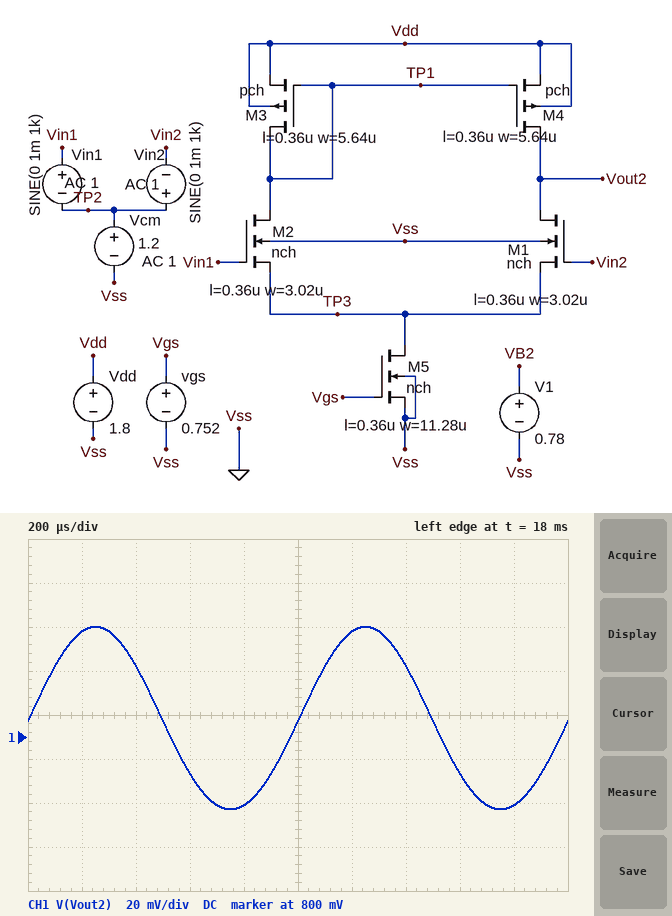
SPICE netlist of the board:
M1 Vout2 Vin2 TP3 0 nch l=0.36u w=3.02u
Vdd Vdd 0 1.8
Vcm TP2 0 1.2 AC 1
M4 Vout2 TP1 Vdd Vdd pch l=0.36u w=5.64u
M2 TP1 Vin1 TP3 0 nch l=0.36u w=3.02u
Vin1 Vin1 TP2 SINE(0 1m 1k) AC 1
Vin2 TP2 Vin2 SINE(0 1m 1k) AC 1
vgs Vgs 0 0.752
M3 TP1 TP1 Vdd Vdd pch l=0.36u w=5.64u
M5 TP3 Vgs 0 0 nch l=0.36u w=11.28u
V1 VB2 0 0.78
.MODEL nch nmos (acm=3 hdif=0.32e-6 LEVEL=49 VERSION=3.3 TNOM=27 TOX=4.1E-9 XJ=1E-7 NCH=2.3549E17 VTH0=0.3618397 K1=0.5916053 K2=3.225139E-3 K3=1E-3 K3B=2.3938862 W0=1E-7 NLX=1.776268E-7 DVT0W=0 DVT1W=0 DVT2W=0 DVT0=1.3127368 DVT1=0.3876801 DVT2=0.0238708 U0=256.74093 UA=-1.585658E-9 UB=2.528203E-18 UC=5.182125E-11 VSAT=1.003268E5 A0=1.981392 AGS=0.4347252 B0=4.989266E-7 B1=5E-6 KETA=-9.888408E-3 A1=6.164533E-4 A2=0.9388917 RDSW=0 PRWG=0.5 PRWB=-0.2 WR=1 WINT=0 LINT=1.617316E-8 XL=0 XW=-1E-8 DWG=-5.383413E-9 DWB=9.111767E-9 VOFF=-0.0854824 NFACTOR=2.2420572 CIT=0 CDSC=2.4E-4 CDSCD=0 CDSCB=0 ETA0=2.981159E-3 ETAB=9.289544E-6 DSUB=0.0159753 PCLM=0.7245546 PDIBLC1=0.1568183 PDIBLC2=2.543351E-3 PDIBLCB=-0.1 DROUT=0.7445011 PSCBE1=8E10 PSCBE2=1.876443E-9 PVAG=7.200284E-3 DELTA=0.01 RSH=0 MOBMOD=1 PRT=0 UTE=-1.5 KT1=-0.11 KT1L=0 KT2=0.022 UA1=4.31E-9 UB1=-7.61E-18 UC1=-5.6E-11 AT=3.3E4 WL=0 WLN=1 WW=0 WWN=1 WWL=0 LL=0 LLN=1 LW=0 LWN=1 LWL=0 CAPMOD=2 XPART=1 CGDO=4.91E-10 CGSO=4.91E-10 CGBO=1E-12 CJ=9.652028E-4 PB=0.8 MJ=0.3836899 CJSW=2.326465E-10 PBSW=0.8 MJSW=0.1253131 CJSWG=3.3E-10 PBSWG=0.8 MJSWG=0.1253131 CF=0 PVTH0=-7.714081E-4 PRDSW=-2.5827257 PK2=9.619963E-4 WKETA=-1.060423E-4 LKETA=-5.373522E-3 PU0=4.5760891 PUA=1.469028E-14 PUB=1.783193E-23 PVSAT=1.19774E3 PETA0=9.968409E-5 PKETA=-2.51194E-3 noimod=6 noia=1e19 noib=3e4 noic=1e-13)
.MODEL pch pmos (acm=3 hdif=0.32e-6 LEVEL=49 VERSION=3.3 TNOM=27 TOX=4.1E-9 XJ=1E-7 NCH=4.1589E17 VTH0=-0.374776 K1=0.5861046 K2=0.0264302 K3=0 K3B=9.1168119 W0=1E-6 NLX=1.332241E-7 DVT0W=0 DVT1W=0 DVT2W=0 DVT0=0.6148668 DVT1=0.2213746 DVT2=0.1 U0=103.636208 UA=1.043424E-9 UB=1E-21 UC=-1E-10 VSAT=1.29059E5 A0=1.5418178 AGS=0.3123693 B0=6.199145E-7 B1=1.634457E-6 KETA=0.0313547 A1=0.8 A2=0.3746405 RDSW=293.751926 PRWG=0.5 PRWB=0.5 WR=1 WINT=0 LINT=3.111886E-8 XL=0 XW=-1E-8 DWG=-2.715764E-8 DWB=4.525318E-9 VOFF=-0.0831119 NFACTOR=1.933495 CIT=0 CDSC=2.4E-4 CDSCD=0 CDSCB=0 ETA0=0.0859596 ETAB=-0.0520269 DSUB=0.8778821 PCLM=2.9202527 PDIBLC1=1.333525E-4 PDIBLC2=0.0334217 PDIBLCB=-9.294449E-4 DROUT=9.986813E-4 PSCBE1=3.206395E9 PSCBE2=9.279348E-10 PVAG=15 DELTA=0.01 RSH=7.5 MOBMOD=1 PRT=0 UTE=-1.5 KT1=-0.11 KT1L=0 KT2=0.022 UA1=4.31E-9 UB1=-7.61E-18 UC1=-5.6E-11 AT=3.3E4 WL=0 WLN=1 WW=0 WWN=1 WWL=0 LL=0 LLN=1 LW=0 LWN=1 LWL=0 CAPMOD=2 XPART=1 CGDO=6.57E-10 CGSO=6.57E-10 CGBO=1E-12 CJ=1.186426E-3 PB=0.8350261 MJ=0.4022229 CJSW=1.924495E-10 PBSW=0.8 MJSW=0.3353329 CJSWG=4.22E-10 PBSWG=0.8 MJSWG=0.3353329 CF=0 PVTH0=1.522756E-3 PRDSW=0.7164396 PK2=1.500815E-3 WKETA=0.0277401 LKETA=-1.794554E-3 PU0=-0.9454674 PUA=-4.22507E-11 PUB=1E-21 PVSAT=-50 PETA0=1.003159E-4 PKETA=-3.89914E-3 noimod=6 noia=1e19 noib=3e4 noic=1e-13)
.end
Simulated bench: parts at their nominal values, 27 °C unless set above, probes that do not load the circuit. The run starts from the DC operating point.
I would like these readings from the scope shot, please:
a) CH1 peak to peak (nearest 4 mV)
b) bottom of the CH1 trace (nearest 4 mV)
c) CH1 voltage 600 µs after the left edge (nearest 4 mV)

84 mV
768 mV
784 mV
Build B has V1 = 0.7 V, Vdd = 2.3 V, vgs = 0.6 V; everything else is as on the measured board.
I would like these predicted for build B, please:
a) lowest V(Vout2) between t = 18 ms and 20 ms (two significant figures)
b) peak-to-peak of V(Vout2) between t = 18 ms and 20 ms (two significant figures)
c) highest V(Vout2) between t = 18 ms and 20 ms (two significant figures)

1.5 V
150 mV
1.7 V
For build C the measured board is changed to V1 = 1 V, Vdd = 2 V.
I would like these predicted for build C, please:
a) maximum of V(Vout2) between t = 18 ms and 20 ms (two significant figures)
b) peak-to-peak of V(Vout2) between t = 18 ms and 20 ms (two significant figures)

1.1 V
100 mV
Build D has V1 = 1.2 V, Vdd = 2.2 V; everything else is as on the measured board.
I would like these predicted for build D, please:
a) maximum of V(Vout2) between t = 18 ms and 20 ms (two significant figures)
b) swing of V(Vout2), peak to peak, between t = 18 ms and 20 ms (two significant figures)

1.3 V
110 mV
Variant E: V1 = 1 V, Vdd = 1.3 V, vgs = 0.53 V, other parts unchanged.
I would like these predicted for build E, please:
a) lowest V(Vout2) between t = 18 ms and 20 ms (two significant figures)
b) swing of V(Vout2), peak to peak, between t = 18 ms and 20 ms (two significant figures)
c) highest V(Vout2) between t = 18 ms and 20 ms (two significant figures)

670 mV
100 mV
770 mV
